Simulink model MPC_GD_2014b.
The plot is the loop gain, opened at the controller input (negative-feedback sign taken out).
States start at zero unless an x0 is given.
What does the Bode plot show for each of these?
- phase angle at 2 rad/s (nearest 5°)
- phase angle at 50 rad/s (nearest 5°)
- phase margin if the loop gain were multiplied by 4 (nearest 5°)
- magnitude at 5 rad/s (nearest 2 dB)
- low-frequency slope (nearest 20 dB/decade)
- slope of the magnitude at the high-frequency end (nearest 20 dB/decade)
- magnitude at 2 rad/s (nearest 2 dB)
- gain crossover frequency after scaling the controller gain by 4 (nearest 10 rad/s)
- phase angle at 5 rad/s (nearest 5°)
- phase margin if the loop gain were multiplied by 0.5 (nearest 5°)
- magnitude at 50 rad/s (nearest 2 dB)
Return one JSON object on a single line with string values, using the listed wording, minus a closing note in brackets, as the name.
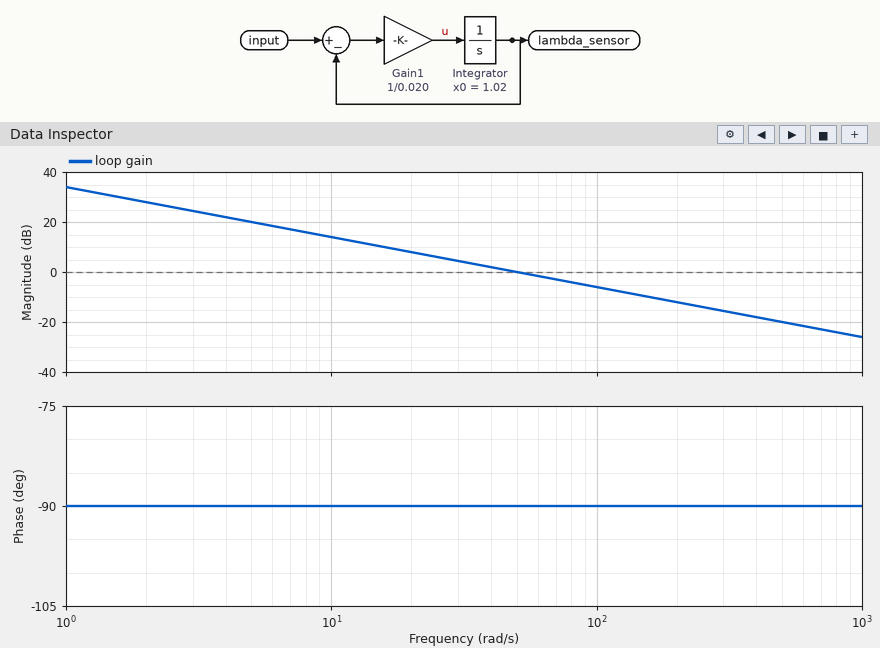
{"phase angle at 2 rad/s": "-90°", "phase angle at 50 rad/s": "-90°", "phase margin if the loop gain were multiplied by 4": "90°", "magnitude at 5 rad/s": "20 dB", "low-frequency slope": "-20 dB/decade", "slope of the magnitude at the high-frequency end": "-20 dB/decade", "magnitude at 2 rad/s": "28 dB", "gain crossover frequency after scaling the controller gain by 4": "200 rad/s", "phase angle at 5 rad/s": "-90°", "phase margin if the loop gain were multiplied by 0.5": "90°", "magnitude at 50 rad/s": "0 dB"}
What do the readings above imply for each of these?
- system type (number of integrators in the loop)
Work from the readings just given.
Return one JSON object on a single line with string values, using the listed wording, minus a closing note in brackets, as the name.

{"system type": "1"}
